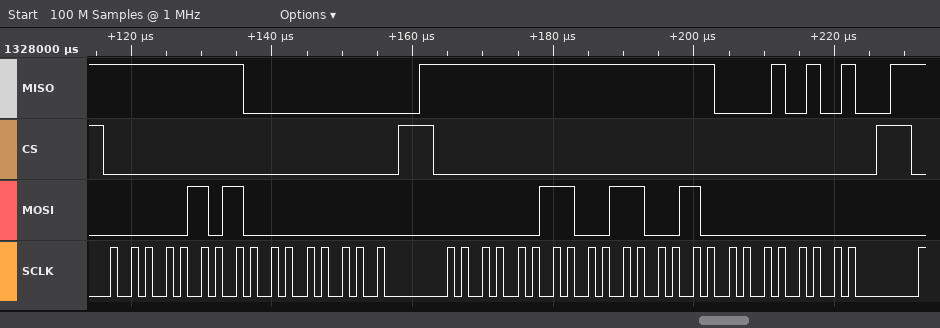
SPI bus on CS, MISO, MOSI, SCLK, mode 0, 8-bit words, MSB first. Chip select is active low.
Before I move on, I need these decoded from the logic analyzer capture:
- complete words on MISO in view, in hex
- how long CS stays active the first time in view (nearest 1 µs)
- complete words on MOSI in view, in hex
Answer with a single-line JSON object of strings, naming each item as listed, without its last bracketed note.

{"complete words on MISO in view, in hex": "FF, 00, FF, FF, 15", "how long CS stays active the first time in view": "42 µs", "complete words on MOSI in view, in hex": "05, 00, 03, 32, 00"}
